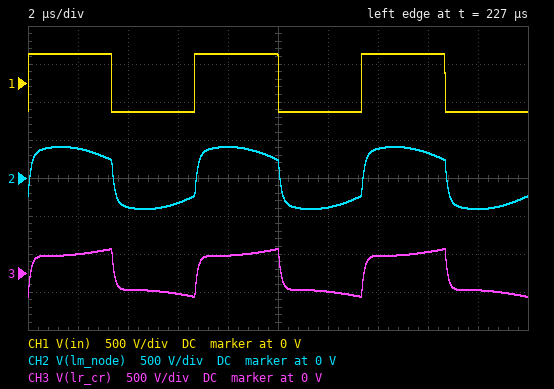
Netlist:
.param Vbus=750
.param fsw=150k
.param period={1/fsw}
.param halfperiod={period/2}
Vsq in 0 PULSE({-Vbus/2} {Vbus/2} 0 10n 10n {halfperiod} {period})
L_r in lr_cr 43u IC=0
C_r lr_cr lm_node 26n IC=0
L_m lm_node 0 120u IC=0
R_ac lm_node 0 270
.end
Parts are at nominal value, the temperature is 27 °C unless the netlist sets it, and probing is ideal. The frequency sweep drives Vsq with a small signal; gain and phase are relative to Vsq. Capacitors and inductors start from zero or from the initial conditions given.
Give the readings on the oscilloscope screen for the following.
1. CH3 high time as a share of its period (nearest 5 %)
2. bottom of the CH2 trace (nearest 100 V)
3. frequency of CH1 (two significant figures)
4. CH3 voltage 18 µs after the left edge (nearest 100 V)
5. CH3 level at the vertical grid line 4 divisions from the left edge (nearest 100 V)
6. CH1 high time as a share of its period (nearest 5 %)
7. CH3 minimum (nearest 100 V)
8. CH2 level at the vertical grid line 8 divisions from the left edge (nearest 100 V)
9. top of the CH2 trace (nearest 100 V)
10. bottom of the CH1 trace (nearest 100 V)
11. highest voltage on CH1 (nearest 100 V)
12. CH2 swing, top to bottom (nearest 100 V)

50 %
-400 V
150 kHz
-200 V
200 V
50 %
-300 V
300 V
400 V
-400 V
400 V
800 V
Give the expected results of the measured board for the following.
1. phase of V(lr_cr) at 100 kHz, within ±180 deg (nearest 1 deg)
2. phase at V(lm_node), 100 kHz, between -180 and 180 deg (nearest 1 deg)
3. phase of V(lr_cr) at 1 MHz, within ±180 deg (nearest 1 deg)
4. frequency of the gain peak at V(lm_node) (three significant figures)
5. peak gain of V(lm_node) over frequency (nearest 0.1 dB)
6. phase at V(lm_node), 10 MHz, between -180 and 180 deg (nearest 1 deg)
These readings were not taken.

-37 deg
13 deg
-37 deg
78.2 kHz
13.4 dB
-82 deg
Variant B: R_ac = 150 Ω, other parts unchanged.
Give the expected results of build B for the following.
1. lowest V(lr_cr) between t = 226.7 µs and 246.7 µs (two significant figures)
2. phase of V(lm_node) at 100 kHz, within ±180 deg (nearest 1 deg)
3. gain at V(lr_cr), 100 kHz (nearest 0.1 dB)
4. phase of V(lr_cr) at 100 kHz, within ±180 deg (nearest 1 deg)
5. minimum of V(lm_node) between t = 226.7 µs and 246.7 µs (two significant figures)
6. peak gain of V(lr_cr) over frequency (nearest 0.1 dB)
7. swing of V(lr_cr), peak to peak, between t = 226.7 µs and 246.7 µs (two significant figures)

-350 V
23 deg
-2.4 dB
-43 deg
-430 V
4.5 dB
690 V
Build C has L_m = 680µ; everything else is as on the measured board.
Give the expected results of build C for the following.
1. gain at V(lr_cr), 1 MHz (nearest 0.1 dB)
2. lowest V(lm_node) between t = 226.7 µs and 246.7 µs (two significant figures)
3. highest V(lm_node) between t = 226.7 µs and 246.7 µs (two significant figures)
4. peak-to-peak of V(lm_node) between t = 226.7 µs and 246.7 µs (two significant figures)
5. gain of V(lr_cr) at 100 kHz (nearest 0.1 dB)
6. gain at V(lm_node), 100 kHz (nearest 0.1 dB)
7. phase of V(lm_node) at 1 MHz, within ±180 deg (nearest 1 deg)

-3.2 dB
-420 V
420 V
840 V
-0.4 dB
0.6 dB
-43 deg
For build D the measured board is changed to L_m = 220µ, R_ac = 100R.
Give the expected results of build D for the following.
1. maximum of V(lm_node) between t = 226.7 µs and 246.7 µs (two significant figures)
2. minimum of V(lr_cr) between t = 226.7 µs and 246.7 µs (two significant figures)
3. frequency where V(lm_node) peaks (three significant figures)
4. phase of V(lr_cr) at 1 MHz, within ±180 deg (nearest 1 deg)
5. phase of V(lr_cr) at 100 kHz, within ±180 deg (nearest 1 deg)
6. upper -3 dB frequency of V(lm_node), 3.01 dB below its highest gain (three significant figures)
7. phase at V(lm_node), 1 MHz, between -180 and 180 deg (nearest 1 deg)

450 V
-400 V
74.5 kHz
-69 deg
-23 deg
168 kHz
-66 deg
